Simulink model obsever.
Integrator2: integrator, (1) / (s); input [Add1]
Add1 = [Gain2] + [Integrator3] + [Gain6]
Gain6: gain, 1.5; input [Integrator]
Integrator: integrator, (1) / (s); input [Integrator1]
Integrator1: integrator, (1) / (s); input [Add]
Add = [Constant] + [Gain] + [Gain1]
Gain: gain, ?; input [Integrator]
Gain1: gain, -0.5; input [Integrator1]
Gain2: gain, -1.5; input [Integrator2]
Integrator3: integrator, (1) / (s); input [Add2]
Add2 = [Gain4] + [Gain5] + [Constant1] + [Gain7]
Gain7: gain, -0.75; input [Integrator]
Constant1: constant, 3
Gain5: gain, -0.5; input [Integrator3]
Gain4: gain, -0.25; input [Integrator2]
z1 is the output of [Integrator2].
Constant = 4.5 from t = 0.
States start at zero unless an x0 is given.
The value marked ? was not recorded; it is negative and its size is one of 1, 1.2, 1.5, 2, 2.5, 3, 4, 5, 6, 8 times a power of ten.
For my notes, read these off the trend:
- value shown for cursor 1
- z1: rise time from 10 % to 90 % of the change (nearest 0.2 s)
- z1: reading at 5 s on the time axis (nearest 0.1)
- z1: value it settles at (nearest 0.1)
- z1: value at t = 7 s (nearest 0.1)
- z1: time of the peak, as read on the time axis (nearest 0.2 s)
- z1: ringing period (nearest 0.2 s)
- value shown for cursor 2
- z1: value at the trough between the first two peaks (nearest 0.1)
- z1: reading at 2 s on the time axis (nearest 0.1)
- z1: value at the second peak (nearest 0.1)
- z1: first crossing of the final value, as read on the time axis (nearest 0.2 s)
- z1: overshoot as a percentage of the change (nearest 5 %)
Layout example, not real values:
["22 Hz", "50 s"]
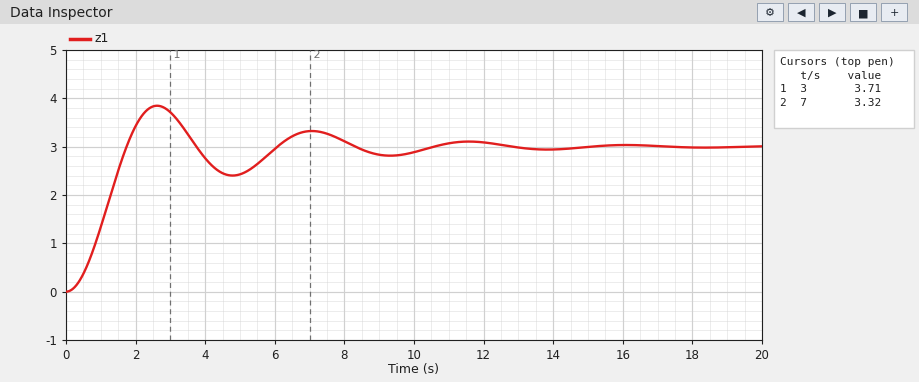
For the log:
["3.71", "1.2 s", "2.4", "3.0", "3.3", "2.6 s", "4.4 s", "3.32", "2.4", "3.4", "3.3", "1.8 s", "30 %"]
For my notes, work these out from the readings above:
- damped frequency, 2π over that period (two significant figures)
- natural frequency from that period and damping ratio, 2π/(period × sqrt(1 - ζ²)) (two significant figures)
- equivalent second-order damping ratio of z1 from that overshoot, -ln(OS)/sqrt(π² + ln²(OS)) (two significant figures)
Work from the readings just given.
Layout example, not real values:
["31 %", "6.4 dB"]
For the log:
["1.4 rad/s", "1.5 rad/s", "0.36"]
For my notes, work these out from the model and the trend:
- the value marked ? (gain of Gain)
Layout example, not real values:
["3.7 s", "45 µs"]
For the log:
["-2"]
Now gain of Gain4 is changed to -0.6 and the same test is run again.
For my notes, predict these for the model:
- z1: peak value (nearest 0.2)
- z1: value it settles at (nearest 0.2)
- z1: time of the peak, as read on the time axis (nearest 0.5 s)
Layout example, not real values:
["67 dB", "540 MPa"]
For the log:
["3.4", "2.2", "2.5 s"]
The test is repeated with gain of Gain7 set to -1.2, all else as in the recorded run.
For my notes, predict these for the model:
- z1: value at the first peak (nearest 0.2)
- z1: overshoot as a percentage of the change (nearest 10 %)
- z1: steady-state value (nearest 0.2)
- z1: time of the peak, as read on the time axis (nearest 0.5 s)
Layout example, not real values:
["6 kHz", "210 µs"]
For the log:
["3.2", "60 %", "2.0", "2.5 s"]
